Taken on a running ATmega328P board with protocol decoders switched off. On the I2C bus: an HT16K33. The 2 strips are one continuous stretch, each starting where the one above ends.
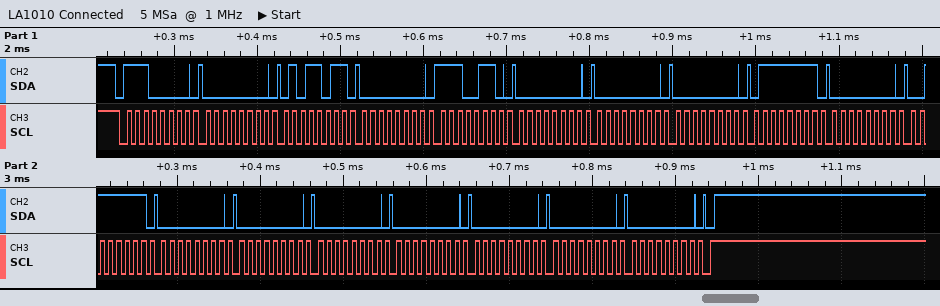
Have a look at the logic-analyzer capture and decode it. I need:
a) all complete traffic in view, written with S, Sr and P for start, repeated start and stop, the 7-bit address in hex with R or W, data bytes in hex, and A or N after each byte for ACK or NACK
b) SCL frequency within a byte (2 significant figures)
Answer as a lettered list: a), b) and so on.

a) S 70W A 00 A 5B A 00 A E6 A 00 A 00 A 00 A 7F A 00 A 3F A 00 A 00 A 00 A 00 A 00 A 00 A 00 A P
b) 100 kHz
